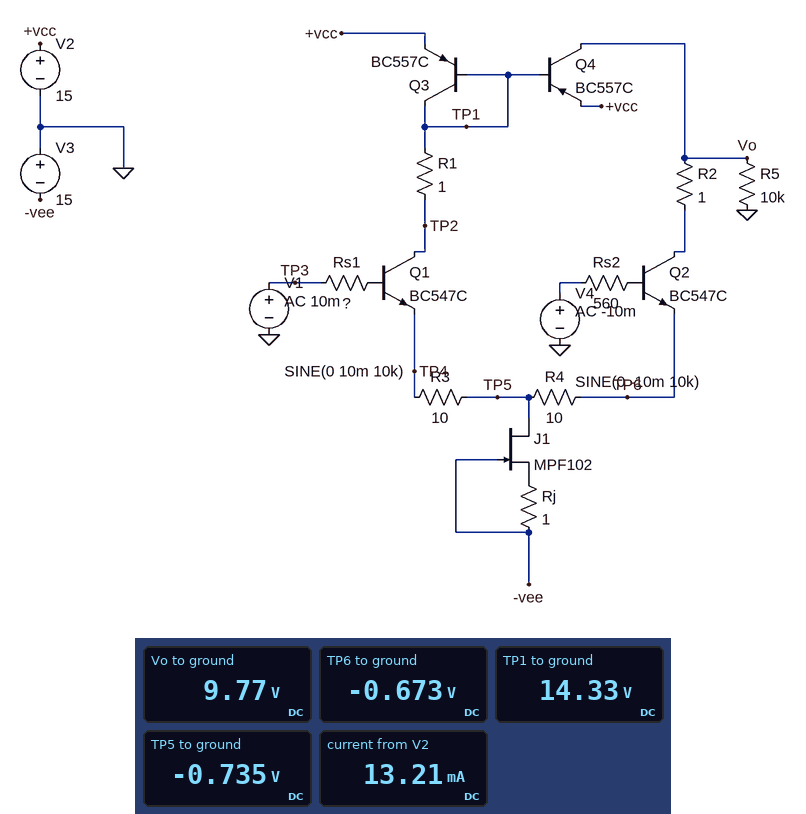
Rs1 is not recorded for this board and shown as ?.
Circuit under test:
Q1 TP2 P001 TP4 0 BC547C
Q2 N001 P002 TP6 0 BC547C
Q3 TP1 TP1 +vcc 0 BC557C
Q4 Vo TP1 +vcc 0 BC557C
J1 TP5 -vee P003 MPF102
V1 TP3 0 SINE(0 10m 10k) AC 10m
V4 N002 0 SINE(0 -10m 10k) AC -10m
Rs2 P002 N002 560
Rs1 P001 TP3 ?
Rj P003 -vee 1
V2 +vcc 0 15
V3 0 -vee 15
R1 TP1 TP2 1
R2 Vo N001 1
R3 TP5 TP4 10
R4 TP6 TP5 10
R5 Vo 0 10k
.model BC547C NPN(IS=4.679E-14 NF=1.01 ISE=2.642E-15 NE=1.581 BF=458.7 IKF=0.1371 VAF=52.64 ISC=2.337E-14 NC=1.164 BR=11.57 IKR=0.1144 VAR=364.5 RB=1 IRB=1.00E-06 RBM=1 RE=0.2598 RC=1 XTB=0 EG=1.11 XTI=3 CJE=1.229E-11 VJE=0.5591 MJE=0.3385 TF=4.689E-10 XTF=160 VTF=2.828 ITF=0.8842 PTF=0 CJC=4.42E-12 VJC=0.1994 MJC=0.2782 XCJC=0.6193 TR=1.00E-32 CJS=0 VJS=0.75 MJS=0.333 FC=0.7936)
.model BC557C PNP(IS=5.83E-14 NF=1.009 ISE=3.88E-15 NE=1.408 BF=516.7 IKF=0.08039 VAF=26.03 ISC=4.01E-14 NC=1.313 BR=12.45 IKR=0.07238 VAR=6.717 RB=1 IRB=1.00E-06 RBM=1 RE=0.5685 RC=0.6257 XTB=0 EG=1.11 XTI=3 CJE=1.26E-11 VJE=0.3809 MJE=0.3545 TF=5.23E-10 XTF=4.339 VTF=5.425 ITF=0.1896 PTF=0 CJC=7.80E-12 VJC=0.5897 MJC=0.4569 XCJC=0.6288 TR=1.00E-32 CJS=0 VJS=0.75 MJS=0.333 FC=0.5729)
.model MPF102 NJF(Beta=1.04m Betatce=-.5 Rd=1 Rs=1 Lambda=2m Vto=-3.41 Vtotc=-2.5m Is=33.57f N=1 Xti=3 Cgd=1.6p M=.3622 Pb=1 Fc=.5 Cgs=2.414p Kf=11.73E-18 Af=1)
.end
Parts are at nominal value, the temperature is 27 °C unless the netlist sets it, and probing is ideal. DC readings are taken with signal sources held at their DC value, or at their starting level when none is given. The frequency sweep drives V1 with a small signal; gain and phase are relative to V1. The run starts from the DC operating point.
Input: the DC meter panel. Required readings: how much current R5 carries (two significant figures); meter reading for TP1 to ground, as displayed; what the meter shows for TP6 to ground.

980 µA
14.33 V
-0.673 V
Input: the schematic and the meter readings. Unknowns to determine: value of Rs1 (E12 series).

820 Ω
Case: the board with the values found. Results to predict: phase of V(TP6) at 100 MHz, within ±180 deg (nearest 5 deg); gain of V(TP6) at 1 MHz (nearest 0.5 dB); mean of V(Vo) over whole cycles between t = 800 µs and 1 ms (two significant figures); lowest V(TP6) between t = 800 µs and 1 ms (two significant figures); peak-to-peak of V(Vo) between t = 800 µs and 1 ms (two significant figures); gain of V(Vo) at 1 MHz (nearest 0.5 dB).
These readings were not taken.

-55 deg
-3.5 dB
9.7 V
-680 mV
7.5 V
41.5 dB
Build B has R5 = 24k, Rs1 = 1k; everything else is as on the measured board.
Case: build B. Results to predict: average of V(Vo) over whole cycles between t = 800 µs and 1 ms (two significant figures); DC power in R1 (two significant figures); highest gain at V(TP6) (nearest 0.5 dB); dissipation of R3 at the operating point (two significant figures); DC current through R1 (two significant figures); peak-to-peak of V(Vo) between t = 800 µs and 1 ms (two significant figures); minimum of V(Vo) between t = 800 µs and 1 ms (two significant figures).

11 V
36 µW
-2.0 dB
360 µW
6.0 mA
8.3 V
6.6 V
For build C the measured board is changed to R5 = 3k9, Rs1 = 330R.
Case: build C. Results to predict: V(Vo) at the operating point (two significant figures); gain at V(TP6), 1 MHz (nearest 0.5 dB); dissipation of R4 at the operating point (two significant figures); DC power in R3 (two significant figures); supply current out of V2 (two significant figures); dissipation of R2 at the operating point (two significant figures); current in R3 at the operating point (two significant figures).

7.5 V
-4.0 dB
350 µW
400 µW
14 mA
35 µW
6.3 mA
